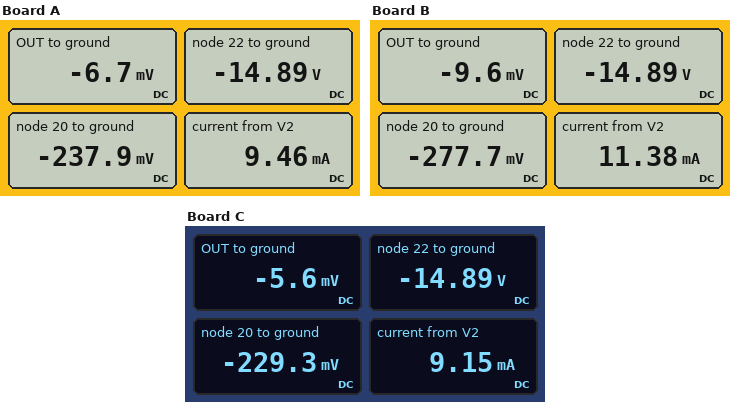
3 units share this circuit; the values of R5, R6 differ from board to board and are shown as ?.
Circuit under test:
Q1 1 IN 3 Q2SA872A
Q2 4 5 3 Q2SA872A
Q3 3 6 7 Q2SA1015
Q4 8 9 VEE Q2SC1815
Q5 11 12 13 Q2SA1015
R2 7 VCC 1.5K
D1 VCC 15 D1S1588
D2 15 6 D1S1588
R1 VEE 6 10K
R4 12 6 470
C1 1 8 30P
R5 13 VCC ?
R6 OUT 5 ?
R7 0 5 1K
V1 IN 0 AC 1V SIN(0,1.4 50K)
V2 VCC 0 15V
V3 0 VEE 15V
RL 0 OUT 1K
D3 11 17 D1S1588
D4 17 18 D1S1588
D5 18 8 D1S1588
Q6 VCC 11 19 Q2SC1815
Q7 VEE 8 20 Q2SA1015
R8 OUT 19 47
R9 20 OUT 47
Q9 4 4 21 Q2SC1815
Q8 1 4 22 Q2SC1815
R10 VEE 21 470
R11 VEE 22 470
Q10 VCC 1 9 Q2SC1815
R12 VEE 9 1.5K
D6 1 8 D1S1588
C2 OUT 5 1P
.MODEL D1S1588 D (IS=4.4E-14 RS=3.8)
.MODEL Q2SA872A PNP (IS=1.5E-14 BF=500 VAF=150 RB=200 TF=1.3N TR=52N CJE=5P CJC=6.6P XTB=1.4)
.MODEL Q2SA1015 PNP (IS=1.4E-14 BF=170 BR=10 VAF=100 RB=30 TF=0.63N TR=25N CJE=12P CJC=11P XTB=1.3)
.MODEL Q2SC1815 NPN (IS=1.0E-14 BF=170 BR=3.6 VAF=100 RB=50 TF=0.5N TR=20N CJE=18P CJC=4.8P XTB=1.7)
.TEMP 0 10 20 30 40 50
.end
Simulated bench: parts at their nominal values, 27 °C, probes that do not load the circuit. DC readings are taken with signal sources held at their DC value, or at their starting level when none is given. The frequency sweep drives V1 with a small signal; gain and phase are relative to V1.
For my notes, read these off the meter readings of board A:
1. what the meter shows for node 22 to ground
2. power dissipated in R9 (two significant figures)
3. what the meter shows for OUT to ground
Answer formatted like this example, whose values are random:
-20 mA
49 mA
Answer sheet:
-14.89 V
1.1 mW
-6.7 mV
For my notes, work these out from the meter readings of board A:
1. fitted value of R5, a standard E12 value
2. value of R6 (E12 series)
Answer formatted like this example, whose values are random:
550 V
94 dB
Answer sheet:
820 Ω
18 kΩ
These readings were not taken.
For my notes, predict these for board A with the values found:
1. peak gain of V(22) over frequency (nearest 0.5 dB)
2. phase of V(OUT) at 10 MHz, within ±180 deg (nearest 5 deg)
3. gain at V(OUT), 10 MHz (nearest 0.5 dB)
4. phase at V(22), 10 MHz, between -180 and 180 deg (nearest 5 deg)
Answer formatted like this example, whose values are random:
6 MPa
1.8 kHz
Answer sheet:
5.0 dB
-155 deg
8.0 dB
-55 deg
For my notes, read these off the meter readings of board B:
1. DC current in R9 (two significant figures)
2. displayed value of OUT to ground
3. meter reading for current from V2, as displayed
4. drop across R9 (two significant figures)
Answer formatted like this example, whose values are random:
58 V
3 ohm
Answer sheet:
5.7 mA
-9.6 mV
11.38 mA
270 mV
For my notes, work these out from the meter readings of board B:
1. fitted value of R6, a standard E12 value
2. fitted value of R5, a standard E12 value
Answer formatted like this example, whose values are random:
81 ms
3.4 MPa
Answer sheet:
27 kΩ
330 Ω
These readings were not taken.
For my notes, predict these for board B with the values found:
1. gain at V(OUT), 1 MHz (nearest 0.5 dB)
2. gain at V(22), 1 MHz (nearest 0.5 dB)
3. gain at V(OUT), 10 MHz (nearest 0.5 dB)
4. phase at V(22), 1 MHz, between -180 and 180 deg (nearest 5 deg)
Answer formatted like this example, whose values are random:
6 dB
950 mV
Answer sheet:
27.5 dB
0.5 dB
7.5 dB
50 deg
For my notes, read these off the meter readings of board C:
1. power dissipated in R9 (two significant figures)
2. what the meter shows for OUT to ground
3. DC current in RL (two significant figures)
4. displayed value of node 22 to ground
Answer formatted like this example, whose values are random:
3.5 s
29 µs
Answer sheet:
1.1 mW
-5.6 mV
5.6 µA
-14.89 V
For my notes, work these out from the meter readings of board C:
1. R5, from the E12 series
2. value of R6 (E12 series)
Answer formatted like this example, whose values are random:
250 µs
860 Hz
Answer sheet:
1 kΩ
15 kΩ
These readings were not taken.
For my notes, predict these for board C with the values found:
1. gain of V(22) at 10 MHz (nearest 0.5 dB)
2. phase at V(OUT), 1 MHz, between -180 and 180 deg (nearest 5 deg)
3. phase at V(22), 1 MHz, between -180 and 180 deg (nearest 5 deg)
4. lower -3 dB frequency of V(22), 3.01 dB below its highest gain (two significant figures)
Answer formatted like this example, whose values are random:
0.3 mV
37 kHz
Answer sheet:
1.0 dB
-25 deg
65 deg
1.9 MHz
